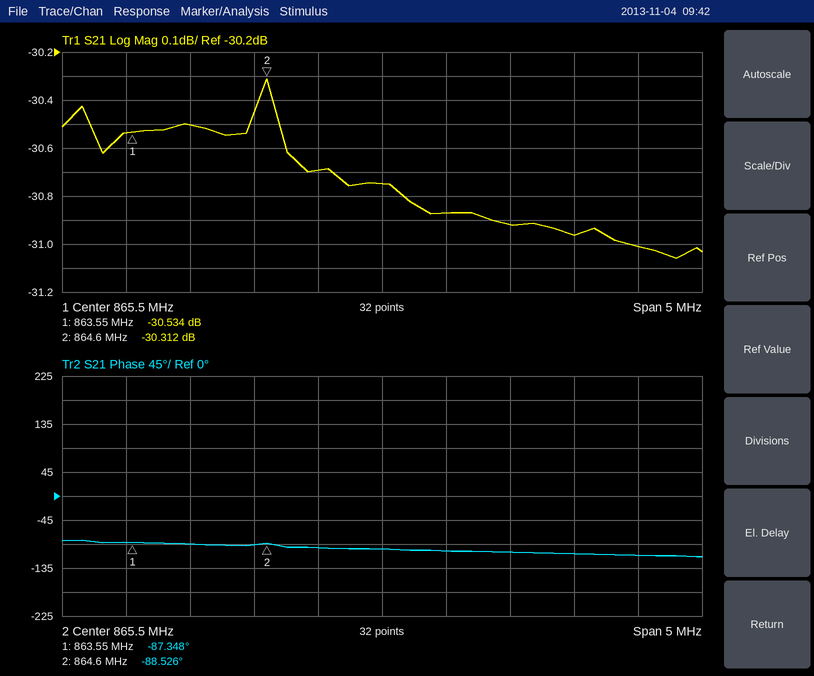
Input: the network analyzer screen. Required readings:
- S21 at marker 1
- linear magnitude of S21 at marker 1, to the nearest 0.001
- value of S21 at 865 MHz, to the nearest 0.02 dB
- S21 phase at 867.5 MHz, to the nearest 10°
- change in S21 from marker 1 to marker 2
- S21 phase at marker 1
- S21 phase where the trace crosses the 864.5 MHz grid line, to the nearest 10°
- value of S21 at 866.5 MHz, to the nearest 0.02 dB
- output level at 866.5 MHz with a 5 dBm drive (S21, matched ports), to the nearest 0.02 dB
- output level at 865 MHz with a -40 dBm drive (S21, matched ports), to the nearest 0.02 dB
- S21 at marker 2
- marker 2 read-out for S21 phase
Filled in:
-30.534 dB
0.030
-30.70 dB
-110°
0.222 dB
-87.348°
-90°
-30.92 dB
-25.92 dBm
-70.70 dBm
-30.312 dB
-88.526°
